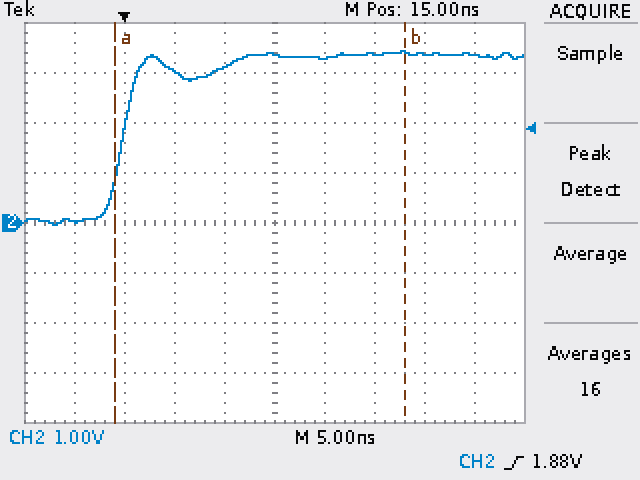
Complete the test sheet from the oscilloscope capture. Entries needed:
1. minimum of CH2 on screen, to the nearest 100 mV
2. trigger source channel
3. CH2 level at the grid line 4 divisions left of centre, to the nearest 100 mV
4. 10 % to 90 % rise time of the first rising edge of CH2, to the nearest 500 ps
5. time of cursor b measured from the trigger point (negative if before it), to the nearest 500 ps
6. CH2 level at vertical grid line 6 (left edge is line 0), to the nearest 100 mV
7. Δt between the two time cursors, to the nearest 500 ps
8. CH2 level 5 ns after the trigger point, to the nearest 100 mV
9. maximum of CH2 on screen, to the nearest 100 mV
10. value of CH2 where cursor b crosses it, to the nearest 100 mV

0.0 V
CH2
0.0 V
3.0 ns
+28.0 ns
3.3 V
29.0 ns
3.0 V
3.4 V
3.4 V
